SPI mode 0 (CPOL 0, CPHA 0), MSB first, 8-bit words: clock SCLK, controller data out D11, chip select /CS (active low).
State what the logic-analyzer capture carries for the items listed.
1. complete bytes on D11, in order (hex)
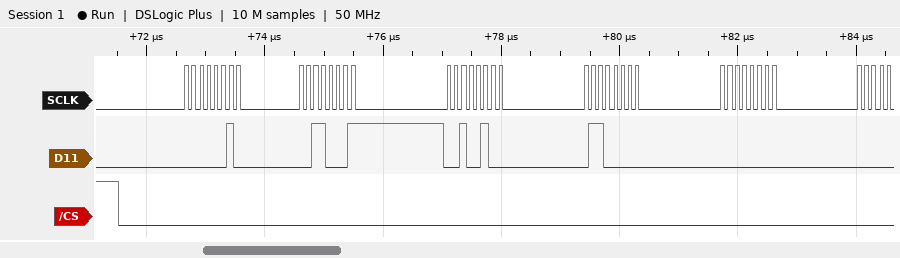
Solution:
02 31 24 60 00
